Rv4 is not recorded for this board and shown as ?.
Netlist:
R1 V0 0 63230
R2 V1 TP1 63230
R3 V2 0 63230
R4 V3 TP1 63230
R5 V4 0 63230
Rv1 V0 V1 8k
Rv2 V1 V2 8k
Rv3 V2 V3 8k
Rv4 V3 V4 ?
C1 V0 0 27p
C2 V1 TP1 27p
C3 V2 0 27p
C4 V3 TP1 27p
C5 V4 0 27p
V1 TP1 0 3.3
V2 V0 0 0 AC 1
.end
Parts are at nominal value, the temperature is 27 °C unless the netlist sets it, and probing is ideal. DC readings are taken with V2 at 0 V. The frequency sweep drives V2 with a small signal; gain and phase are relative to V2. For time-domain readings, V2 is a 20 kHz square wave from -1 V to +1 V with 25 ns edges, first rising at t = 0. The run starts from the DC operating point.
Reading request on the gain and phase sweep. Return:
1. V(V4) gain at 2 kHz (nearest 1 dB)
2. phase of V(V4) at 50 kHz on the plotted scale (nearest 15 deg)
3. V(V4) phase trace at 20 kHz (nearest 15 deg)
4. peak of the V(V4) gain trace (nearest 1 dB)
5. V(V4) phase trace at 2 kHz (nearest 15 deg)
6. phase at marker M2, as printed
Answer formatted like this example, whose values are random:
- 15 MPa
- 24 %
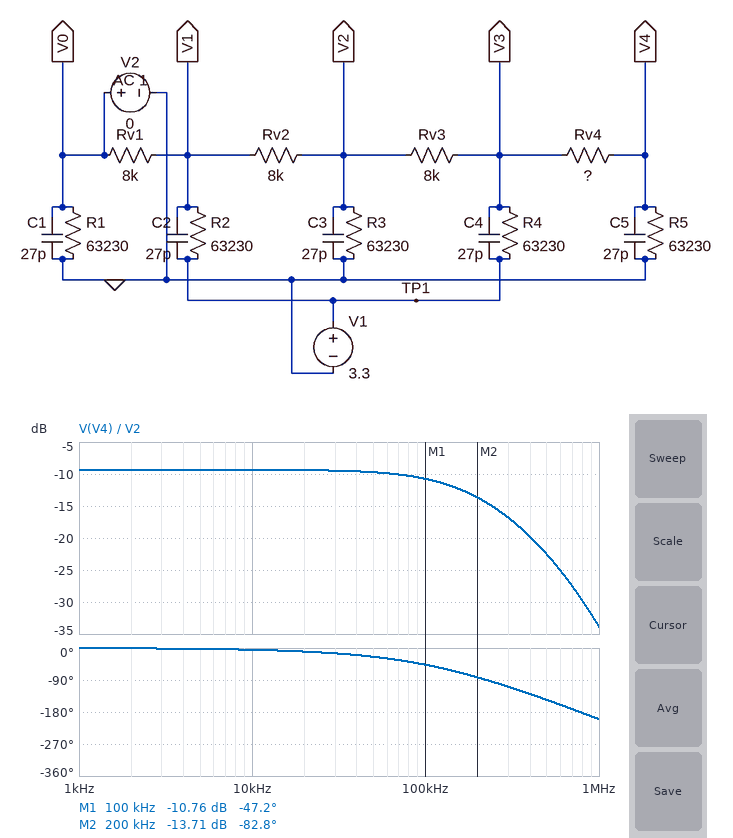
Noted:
- -9 dB
- -30 deg
- -15 deg
- -9 dB
- 0 deg
- -82.8 deg
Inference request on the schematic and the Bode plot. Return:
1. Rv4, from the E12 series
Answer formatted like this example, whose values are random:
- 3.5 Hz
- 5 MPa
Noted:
- 22 kΩ
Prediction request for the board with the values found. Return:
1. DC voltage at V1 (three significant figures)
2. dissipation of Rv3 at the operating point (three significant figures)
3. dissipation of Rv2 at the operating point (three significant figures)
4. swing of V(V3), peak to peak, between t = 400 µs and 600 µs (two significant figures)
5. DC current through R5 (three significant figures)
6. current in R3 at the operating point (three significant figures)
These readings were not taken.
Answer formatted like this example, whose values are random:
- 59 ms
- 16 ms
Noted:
- 499 mV
- 6.38 µW
- 2.61 µW
- 920 mV
- 10.2 µA
- 10.2 µA
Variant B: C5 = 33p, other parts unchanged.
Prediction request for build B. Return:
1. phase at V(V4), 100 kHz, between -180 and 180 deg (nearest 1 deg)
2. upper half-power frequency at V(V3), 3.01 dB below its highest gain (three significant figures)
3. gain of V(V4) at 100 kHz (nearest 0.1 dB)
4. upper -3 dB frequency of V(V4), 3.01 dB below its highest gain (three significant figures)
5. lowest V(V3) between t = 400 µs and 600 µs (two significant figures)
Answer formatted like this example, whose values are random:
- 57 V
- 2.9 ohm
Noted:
- -51 deg
- 179 kHz
- -11.1 dB
- 140 kHz
- 410 mV
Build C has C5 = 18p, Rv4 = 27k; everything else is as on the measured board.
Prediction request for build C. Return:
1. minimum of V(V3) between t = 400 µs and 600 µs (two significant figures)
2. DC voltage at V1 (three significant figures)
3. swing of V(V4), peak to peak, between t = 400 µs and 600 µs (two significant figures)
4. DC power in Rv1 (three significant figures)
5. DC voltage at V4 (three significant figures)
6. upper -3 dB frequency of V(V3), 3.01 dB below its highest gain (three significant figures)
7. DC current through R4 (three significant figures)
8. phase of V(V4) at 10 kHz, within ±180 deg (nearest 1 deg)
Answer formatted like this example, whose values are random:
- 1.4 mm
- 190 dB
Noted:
- 410 mV
- 501 mV
- 650 mV
- 31.4 µW
- 614 mV
- 213 kHz
- 38.3 µA
- -4 deg
